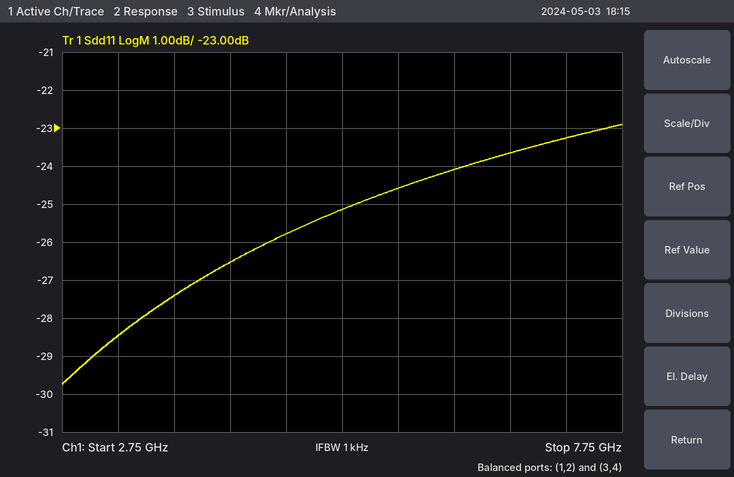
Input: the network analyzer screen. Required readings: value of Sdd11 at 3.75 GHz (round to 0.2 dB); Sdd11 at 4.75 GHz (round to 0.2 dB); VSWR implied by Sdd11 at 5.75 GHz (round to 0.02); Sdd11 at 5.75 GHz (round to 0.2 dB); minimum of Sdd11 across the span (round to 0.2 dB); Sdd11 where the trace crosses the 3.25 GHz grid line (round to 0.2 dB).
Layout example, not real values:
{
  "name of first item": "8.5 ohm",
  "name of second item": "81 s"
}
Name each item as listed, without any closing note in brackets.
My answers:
{
  "value of Sdd11 at 3.75 GHz": "-27.4 dB",
  "Sdd11 at 4.75 GHz": "-25.8 dB",
  "VSWR implied by Sdd11 at 5.75 GHz": "1.12",
  "Sdd11 at 5.75 GHz": "-24.6 dB",
  "minimum of Sdd11 across the span": "-29.8 dB",
  "Sdd11 where the trace crosses the 3.25 GHz grid line": "-28.4 dB"
}
